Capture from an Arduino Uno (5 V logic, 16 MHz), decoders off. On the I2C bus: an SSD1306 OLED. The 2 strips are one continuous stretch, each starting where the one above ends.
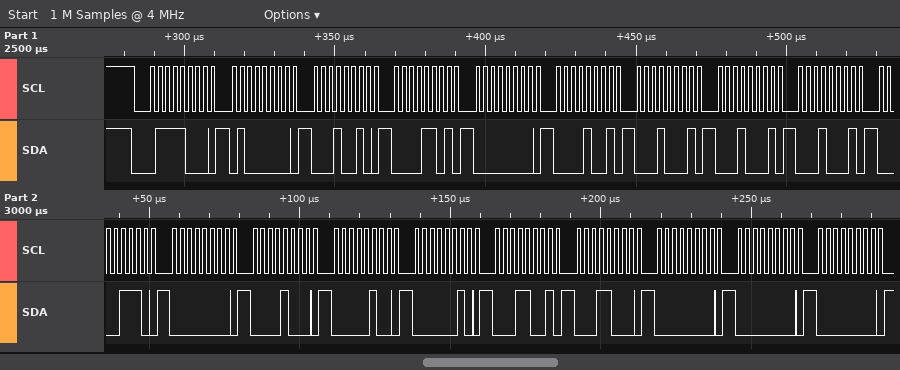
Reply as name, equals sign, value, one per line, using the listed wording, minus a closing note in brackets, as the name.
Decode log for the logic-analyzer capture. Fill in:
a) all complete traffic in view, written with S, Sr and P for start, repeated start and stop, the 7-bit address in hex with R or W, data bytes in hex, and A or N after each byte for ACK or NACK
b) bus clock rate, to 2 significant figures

all complete traffic in view, written with S, Sr and P for start, repeated start and stop, the 7-bit address in hex with R or W, data bytes in hex, and A or N after each byte for ACK or NACK = S 3CW A 40 A 12 A 0D A 00 A 09 A 11 A 11 A 11 A 0E A 00 A 08 A 04 A 02 A 19 A 18 A 00 A 00 A 00 A
bus clock rate, to 2 significant figures = 400 kHz
